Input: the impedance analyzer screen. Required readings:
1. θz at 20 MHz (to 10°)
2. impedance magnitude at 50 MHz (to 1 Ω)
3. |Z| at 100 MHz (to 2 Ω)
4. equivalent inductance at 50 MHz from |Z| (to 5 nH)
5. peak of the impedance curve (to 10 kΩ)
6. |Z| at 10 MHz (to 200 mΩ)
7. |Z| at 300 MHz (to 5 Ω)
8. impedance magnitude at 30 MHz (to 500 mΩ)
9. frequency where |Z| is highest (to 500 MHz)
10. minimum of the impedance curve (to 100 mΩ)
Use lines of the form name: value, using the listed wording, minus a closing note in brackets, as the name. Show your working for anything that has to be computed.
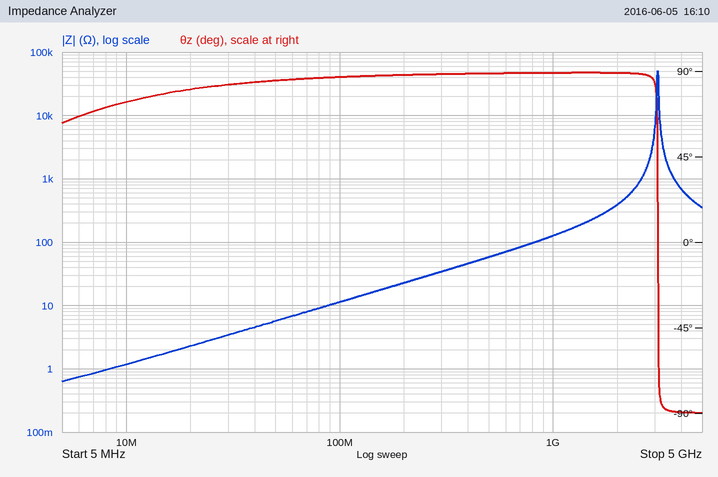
θz at 20 MHz: 80°
impedance magnitude at 50 MHz: 6 Ω
|Z| at 100 MHz: 12 Ω
equivalent inductance at 50 MHz from |Z|: L = 6 Ω/(2π × 50 MHz) ≈ 19.1 nH, so 20 nH to the nearest 5 nH
peak of the impedance curve: 50 kΩ
|Z| at 10 MHz: 1.2 Ω
|Z| at 300 MHz: 35 Ω
impedance magnitude at 30 MHz: 3.5 Ω
frequency where |Z| is highest: 3.0 GHz
minimum of the impedance curve: 600 mΩ
